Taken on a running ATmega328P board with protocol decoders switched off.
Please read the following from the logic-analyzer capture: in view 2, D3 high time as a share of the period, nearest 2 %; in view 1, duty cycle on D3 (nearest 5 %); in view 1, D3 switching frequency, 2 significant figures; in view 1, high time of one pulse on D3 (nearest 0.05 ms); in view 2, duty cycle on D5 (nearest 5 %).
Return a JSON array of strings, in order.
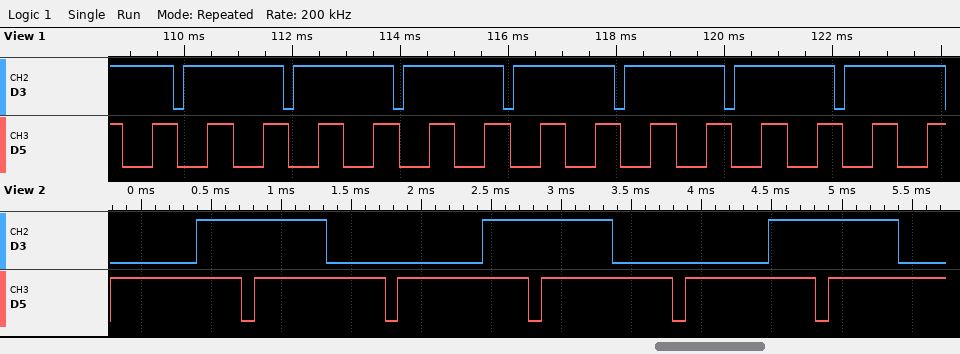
["46 %", "90 %", "490 Hz", "1.85 ms", "90 %"]
